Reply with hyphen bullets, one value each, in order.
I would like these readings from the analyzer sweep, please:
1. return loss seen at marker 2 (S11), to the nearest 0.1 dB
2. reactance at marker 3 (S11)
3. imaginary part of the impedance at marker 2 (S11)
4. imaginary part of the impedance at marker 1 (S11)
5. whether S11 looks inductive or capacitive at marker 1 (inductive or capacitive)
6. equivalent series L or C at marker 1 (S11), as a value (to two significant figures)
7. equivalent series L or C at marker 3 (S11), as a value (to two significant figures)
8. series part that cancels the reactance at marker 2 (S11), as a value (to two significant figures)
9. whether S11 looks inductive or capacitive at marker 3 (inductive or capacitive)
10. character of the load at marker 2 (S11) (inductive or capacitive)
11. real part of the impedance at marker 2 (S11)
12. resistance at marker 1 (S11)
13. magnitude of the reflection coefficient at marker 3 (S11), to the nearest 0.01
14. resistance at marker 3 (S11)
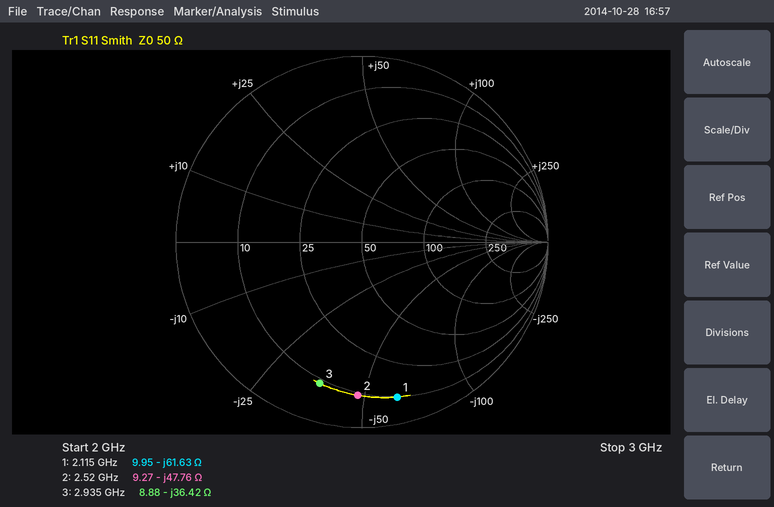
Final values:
- 1.7 dB
- -36.42 Ω
- -47.76 Ω
- -61.63 Ω
- capacitive
- 1.2 pF
- 1.5 pF
- 3.0 nH
- capacitive
- capacitive
- 9.27 Ω
- 9.95 Ω
- 0.79
- 8.88 Ω
